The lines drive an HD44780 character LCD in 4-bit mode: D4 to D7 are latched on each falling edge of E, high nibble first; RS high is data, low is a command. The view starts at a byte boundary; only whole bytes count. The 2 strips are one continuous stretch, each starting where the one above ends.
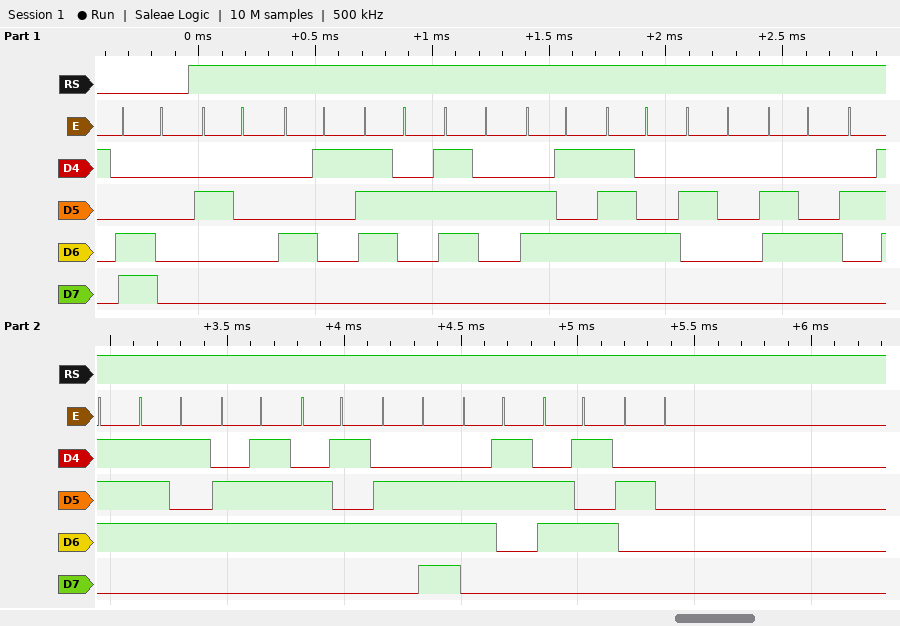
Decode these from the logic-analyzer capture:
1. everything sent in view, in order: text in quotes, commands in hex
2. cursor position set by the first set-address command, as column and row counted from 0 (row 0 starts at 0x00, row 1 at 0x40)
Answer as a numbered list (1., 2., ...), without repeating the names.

1. 0xC0 " Arret d'ugence "
2. column 0, row 1
